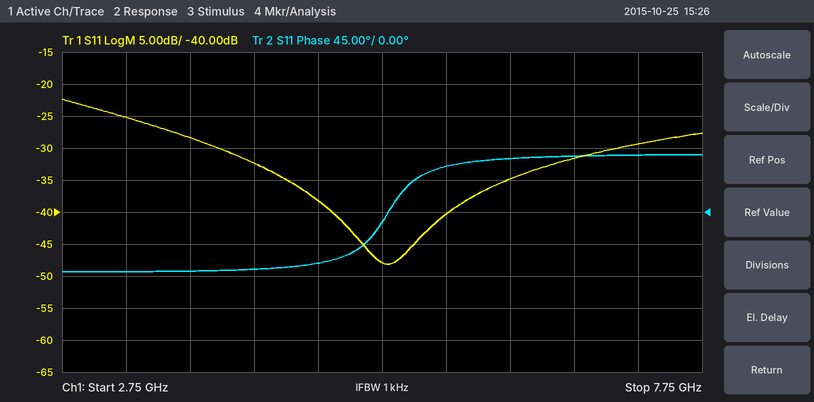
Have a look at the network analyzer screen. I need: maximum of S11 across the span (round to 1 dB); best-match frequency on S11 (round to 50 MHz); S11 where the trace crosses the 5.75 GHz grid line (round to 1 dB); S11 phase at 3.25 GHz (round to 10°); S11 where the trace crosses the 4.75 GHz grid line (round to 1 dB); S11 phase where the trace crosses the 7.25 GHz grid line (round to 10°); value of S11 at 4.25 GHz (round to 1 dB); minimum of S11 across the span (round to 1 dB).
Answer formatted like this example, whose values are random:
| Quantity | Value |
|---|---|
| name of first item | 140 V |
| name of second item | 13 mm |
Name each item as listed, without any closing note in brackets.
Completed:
| Quantity | Value |
|---|---|
| maximum of S11 across the span | -22 dB |
| best-match frequency on S11 | 5.30 GHz |
| S11 where the trace crosses the 5.75 GHz grid line | -40 dB |
| S11 phase at 3.25 GHz | -80° |
| S11 where the trace crosses the 4.75 GHz grid line | -38 dB |
| S11 phase where the trace crosses the 7.25 GHz grid line | 80° |
| value of S11 at 4.25 GHz | -32 dB |
| minimum of S11 across the span | -48 dB |
